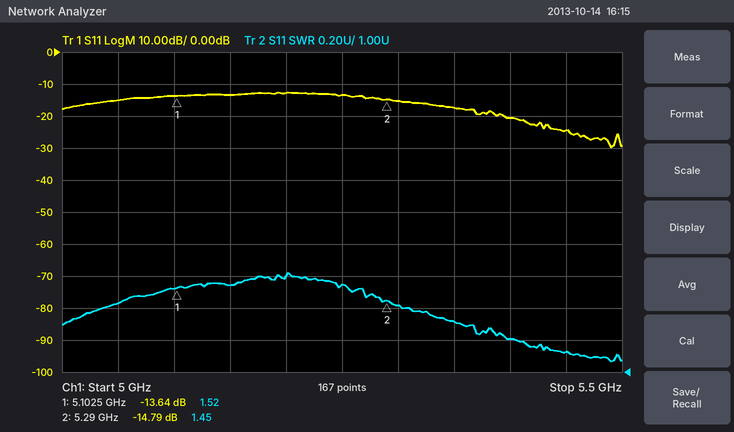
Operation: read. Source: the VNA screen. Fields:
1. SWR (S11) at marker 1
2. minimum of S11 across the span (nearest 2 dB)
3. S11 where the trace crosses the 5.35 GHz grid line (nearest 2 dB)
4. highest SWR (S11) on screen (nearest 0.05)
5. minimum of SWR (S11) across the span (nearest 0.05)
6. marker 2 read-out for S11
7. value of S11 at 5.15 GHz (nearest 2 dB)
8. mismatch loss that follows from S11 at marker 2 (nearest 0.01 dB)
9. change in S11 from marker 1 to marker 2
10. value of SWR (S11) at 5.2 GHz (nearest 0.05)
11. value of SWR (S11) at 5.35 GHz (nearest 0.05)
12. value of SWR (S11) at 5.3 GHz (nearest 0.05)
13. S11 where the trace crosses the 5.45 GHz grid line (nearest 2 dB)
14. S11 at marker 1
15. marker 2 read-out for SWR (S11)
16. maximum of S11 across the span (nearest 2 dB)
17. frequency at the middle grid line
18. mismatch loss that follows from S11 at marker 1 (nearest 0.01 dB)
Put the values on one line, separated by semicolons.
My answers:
1.52; -30 dB; -18 dB; 1.60; 1.05; -14.79 dB; -14 dB; 0.15 dB; -1.15 dB; 1.60; 1.30; 1.40; -24 dB; -13.64 dB; 1.45; -12 dB; 5.25 GHz; 0.19 dB
